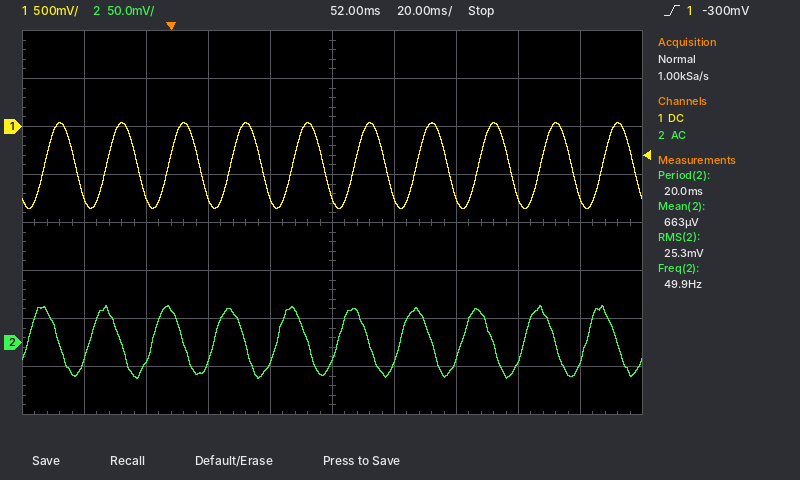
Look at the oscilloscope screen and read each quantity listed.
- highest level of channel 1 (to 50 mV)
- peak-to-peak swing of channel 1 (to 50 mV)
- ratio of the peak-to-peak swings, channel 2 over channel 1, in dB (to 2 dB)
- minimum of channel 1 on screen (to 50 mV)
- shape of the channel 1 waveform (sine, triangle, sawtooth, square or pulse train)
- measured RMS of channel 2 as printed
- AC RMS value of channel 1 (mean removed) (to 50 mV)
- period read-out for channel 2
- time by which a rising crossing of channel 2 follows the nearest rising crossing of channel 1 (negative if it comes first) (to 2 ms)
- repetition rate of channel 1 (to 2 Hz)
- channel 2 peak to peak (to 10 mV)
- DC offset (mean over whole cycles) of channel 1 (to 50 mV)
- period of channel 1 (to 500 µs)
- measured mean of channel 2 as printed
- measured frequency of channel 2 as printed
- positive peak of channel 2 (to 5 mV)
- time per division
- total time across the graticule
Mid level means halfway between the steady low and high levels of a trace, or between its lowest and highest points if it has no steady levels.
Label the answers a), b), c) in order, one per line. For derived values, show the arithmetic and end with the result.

a) 50 mV
b) 50 mV − (-850 mV) = 900 mV
c) 20 log10(80 mV / 900 mV) ≈ -21.0 dB, so -22 dB to the nearest 2 dB
d) -850 mV
e) sine
f) 25.3 mV
g) 900 mV / (2√2) ≈ 318 mV, so 300 mV to the nearest 50 mV
h) 20.0 ms
i) -6 ms
j) 1 / 20.0 ms ≈ 50 Hz
k) 80 mV
l) (50 mV + (-850 mV)) / 2 ≈ -400 mV
m) 20.0 ms
n) 663 µV
o) 49.9 Hz
p) 40 mV
q) 20 ms
r) 200 ms
